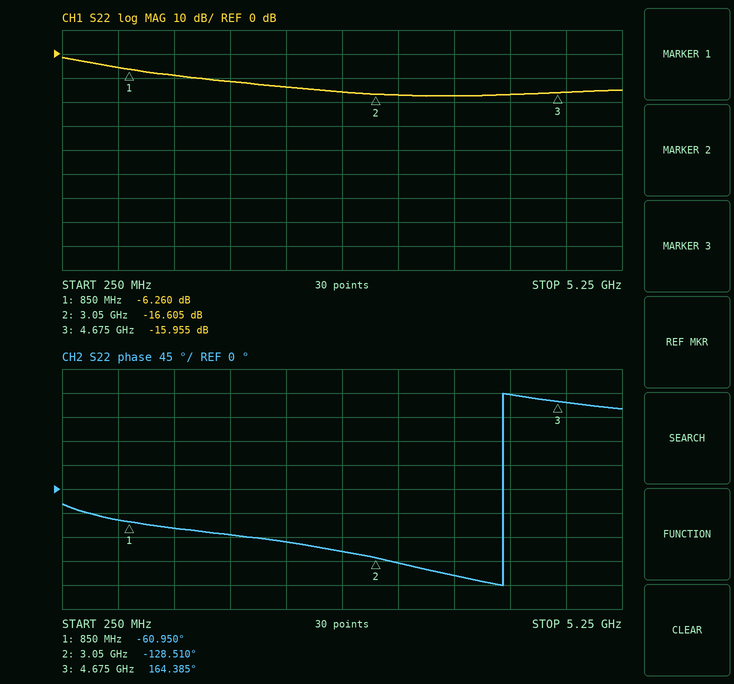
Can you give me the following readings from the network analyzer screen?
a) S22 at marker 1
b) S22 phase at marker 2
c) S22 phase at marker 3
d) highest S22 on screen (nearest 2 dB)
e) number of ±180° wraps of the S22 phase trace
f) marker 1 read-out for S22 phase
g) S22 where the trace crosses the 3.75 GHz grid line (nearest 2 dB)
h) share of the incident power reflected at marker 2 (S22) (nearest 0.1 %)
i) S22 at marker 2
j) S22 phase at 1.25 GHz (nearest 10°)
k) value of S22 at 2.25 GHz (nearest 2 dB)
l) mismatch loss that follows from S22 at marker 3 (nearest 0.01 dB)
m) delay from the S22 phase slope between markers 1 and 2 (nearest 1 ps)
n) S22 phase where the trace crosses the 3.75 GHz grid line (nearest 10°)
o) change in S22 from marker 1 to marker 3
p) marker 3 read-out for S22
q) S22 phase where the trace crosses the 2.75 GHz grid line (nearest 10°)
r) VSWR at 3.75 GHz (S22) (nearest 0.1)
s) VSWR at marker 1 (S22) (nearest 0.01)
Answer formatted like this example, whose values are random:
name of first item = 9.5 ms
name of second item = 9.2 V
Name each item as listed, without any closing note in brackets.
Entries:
S22 at marker 1 = -6.260 dB
S22 phase at marker 2 = -128.510°
S22 phase at marker 3 = 164.385°
highest S22 on screen = -2 dB
number of ±180° wraps of the S22 phase trace = 1
marker 1 read-out for S22 phase = -60.950°
S22 where the trace crosses the 3.75 GHz grid line = -18 dB
share of the incident power reflected at marker 2 (S22) = 2.2 %
S22 at marker 2 = -16.605 dB
S22 phase at 1.25 GHz = -70°
value of S22 at 2.25 GHz = -14 dB
mismatch loss that follows from S22 at marker 3 = 0.11 dB
delay from the S22 phase slope between markers 1 and 2 = 85 ps
S22 phase where the trace crosses the 3.75 GHz grid line = -160°
change in S22 from marker 1 to marker 3 = -9.695 dB
marker 3 read-out for S22 = -15.955 dB
S22 phase where the trace crosses the 2.75 GHz grid line = -120°
VSWR at 3.75 GHz (S22) = 1.3
VSWR at marker 1 (S22) = 2.89
